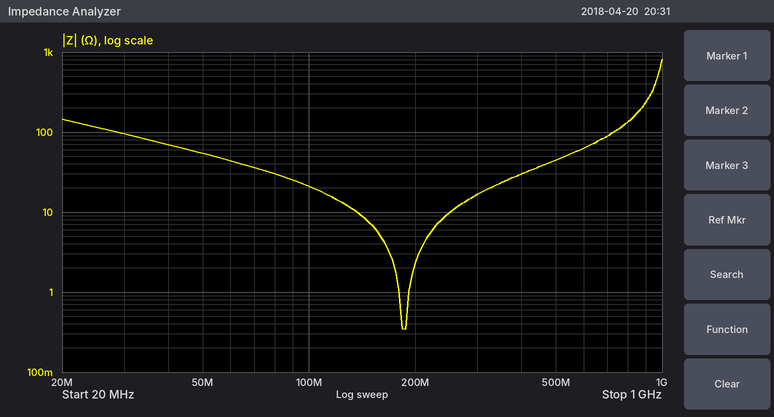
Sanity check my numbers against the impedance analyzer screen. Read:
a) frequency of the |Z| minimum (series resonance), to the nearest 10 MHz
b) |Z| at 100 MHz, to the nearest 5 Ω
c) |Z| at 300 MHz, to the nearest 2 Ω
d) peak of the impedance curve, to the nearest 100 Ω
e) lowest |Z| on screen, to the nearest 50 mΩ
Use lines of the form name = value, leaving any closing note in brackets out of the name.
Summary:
frequency of the |Z| minimum (series resonance), to the nearest 10 MHz = 190 MHz
|Z| at 100 MHz, to the nearest 5 Ω = 20 Ω
|Z| at 300 MHz, to the nearest 2 Ω = 16 Ω
peak of the impedance curve, to the nearest 100 Ω = 800 Ω
lowest |Z| on screen, to the nearest 50 mΩ = 350 mΩ
